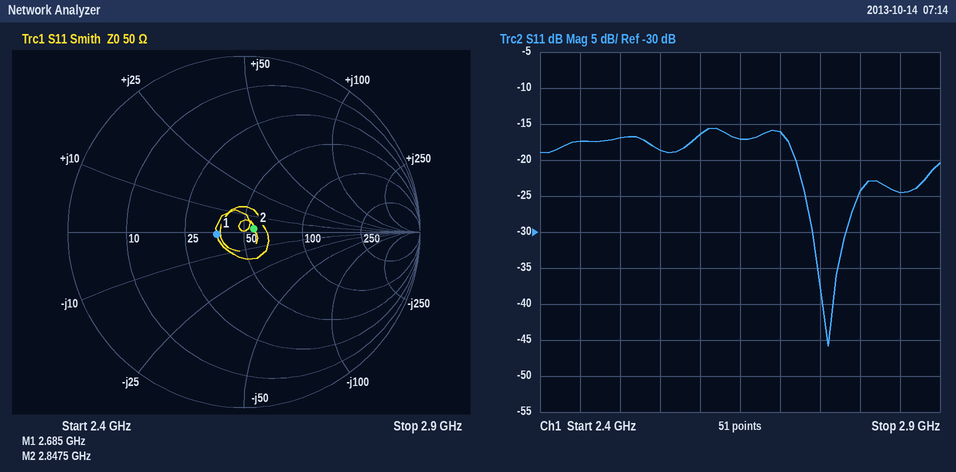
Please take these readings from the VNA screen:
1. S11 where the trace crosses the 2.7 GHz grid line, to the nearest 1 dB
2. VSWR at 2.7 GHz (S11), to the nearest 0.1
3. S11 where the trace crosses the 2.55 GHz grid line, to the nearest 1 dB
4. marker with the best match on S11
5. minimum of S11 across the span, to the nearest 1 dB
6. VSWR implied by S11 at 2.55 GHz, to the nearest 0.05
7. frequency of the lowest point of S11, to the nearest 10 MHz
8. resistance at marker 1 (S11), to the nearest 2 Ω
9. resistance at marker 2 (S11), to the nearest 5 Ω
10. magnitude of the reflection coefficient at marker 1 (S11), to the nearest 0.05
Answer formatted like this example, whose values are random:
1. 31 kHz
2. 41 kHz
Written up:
1. -16 dB
2. 1.4
3. -19 dB
4. marker 2
5. -46 dB
6. 1.25
7. 2.76 GHz
8. 36 Ω
9. 55 Ω
10. 0.15
